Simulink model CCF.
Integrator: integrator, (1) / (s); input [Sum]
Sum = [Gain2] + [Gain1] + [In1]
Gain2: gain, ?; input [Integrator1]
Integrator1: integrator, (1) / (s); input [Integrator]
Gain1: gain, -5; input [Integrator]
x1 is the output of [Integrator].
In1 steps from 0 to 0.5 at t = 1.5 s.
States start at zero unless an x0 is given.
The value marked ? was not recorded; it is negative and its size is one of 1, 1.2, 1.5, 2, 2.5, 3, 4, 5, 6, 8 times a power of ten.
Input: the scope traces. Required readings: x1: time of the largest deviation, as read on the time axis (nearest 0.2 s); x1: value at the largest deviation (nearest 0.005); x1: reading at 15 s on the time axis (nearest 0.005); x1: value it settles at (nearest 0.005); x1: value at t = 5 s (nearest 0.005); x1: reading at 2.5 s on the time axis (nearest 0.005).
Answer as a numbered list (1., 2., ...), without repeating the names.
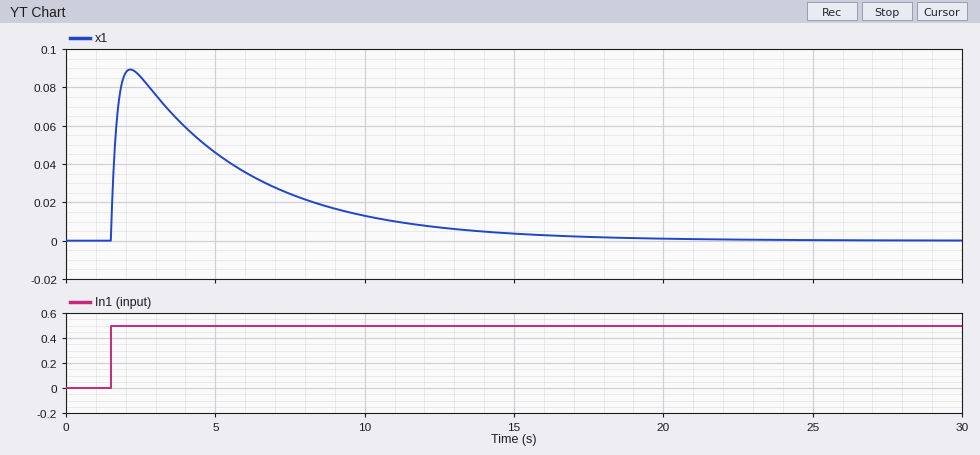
1. 2.2 s
2. 0.090
3. 0.005
4. 0.000
5. 0.045
6. 0.085
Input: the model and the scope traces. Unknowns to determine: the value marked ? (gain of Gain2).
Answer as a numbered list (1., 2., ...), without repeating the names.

1. -1.2
